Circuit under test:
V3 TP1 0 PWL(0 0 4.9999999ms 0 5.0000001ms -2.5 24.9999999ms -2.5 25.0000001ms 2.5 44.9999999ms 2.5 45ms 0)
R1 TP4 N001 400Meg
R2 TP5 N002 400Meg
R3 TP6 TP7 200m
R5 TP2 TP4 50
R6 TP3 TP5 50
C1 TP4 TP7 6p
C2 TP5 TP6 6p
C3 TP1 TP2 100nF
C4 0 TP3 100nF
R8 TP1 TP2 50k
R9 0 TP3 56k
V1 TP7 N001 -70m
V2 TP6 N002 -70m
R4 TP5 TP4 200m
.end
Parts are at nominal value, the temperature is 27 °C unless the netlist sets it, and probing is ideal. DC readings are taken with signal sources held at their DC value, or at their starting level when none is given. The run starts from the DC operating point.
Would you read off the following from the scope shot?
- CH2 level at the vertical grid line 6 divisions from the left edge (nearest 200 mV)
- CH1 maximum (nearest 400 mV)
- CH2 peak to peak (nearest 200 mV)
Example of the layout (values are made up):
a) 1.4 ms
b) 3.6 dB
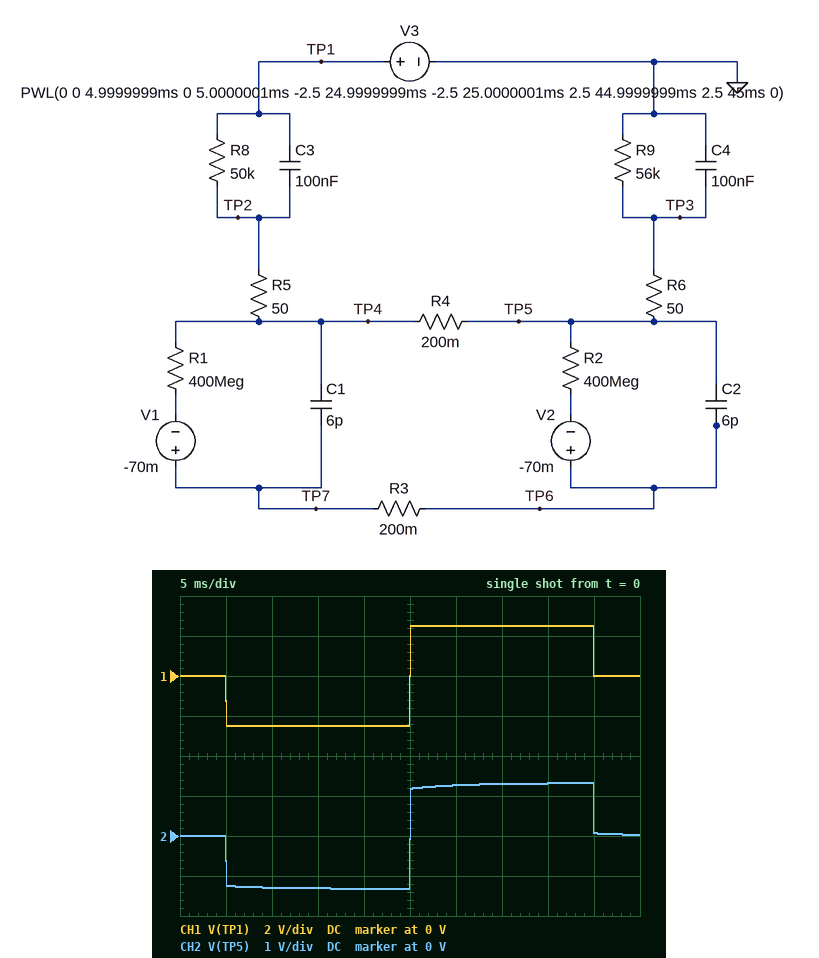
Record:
a) 1.2 V
b) 2.4 V
c) 2.6 V
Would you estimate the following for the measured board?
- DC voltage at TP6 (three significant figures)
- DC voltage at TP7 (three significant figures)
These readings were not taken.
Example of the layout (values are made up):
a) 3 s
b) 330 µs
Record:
a) -70.0 mV
b) -70.0 mV
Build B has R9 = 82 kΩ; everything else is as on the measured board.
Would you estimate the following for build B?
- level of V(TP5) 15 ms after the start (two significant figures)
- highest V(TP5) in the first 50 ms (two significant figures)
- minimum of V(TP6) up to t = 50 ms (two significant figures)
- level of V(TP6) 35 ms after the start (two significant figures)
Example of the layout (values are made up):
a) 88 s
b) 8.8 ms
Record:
a) -1.5 V
b) 1.5 V
c) -1.6 V
d) 1.4 V
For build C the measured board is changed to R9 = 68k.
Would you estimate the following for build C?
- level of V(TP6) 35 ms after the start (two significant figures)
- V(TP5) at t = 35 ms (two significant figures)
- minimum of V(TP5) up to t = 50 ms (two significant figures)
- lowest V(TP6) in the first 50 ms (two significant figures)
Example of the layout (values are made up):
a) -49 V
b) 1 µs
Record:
a) 1.3 V
b) 1.4 V
c) -1.4 V
d) -1.5 V
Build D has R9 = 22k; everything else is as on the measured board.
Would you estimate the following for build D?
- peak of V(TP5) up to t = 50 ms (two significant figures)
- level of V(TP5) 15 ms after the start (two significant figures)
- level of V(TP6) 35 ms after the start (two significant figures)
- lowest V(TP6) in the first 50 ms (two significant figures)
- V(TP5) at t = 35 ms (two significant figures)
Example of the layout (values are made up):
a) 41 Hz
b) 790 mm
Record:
a) 1.7 V
b) -780 mV
c) 730 mV
d) -1.3 V
e) 800 mV
